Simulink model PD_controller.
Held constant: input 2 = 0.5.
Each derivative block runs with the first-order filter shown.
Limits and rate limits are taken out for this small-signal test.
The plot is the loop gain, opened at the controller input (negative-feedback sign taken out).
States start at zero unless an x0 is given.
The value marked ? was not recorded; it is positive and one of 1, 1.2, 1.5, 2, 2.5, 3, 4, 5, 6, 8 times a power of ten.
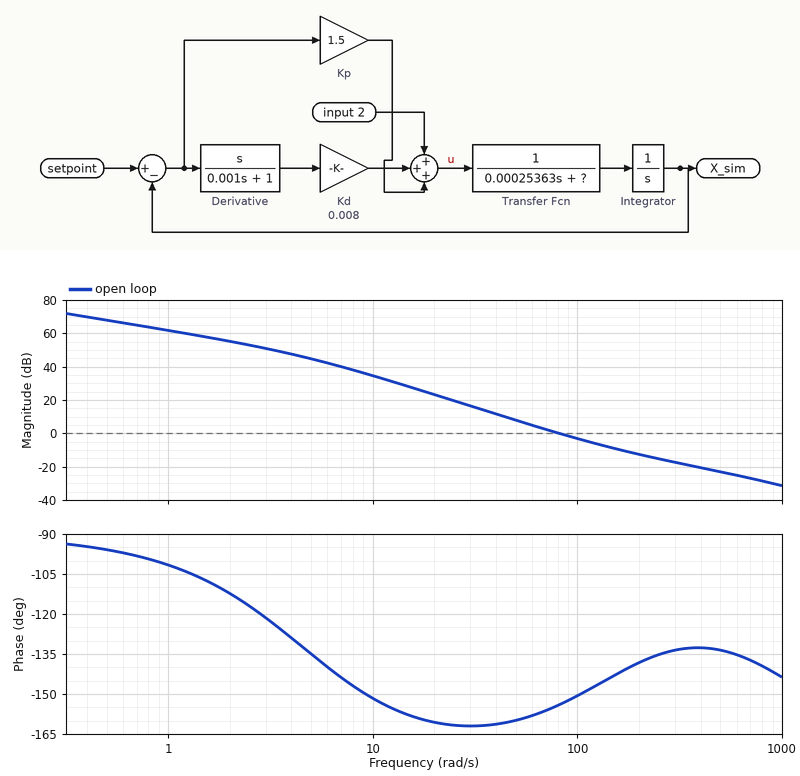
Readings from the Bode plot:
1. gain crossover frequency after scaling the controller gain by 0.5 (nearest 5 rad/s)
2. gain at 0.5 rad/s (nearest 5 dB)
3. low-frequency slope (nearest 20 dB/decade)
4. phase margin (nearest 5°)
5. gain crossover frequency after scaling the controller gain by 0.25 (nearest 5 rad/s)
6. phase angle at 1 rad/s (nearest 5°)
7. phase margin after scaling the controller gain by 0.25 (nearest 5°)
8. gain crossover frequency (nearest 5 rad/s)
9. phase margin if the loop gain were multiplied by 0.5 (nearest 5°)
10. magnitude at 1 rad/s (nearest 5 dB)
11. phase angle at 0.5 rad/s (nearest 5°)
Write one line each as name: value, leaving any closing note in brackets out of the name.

gain crossover frequency after scaling the controller gain by 0.5: 55 rad/s
gain at 0.5 rad/s: 70 dB
low-frequency slope: -20 dB/decade
phase margin: 25°
gain crossover frequency after scaling the controller gain by 0.25: 40 rad/s
phase angle at 1 rad/s: -100°
phase margin after scaling the controller gain by 0.25: 20°
gain crossover frequency: 80 rad/s
phase margin if the loop gain were multiplied by 0.5: 20°
magnitude at 1 rad/s: 60 dB
phase angle at 0.5 rad/s: -95°
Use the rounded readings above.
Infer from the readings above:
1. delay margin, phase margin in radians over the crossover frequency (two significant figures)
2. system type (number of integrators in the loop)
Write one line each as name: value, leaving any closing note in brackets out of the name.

delay margin, phase margin in radians over the crossover frequency: 0.0055 s
system type: 1
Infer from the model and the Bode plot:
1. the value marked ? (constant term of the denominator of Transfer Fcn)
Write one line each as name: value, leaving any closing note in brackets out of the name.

the value marked ?: 0.0012
